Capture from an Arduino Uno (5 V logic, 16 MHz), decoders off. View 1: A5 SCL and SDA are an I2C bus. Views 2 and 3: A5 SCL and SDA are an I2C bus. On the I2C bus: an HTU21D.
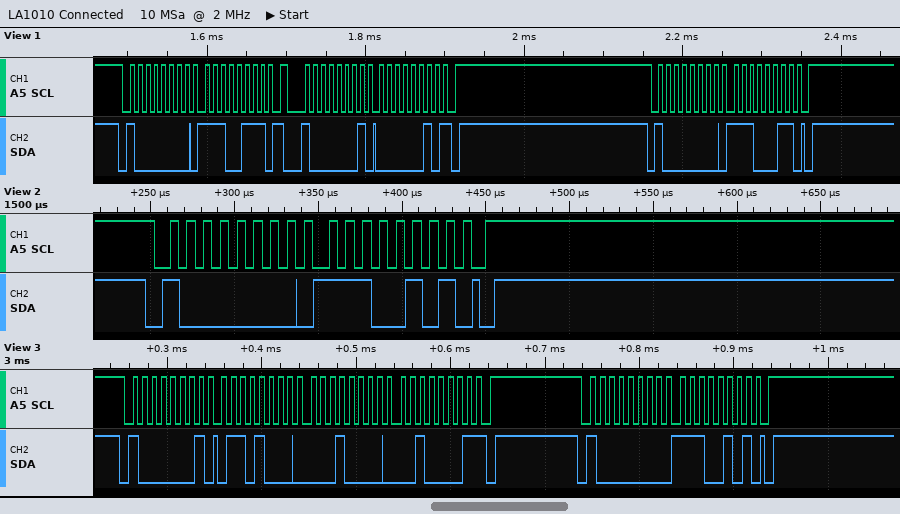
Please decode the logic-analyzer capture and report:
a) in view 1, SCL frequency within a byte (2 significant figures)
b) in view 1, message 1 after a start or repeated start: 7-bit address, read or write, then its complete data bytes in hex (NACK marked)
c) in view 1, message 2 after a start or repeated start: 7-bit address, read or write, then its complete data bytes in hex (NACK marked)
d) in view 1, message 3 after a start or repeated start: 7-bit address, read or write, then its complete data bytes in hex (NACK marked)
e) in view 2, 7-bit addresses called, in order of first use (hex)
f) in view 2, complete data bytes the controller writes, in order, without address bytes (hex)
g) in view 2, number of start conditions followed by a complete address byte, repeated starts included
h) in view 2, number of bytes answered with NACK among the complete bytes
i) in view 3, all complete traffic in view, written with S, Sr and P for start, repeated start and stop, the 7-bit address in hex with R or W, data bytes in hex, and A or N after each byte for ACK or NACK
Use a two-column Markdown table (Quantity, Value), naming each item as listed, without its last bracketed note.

| Quantity | Value |
|---|---|
| in view 1, SCL frequency within a byte | 100 kHz |
| in view 1, message 1 after a start or repeated start: 7-bit address, read or write, then its complete data bytes in hex | 0x40 write: E7 |
| in view 1, message 2 after a start or repeated start: 7-bit address, read or write, then its complete data bytes in hex | 0x40 read: 02 NACK |
| in view 1, message 3 after a start or repeated start: 7-bit address, read or write, then its complete data bytes in hex | 0x40 write: E3 |
| in view 2, 7-bit addresses called, in order of first use | 0x40 |
| in view 2, complete data bytes the controller writes, in order, without address bytes | E5 |
| in view 2, number of start conditions followed by a complete address byte, repeated starts included | 1 |
| in view 2, number of bytes answered with NACK among the complete bytes | 0 |
| in view 3, all complete traffic in view, written with S, Sr and P for start, repeated start and stop, the 7-bit address in hex with R or W, data bytes in hex, and A or N after each byte for ACK or NACK | S 40R A 68 A 10 A 21 N P S 40W A E5 A P |
